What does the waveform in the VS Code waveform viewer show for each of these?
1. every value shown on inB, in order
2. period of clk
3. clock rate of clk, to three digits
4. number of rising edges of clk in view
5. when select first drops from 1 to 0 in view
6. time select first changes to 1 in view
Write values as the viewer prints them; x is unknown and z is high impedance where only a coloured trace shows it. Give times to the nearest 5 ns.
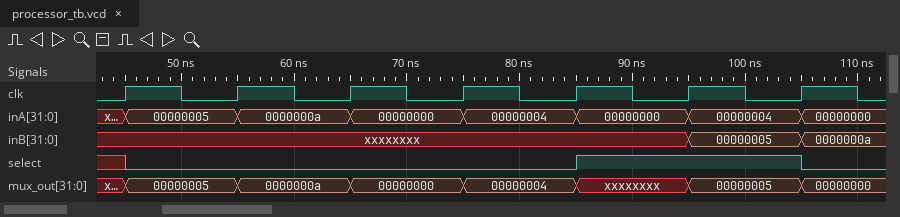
xxxxxxxx, 00000005, 0000000a
10 ns
100 MHz
7
105 ns
85 ns
